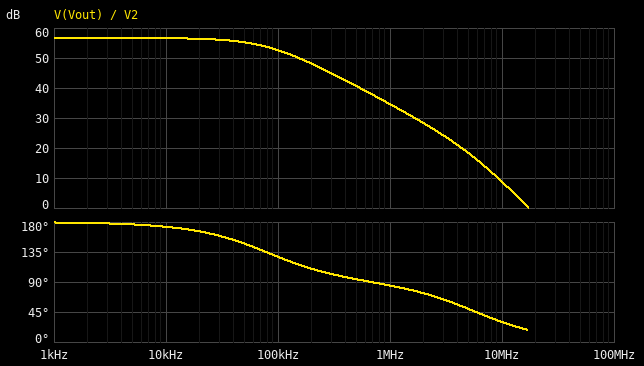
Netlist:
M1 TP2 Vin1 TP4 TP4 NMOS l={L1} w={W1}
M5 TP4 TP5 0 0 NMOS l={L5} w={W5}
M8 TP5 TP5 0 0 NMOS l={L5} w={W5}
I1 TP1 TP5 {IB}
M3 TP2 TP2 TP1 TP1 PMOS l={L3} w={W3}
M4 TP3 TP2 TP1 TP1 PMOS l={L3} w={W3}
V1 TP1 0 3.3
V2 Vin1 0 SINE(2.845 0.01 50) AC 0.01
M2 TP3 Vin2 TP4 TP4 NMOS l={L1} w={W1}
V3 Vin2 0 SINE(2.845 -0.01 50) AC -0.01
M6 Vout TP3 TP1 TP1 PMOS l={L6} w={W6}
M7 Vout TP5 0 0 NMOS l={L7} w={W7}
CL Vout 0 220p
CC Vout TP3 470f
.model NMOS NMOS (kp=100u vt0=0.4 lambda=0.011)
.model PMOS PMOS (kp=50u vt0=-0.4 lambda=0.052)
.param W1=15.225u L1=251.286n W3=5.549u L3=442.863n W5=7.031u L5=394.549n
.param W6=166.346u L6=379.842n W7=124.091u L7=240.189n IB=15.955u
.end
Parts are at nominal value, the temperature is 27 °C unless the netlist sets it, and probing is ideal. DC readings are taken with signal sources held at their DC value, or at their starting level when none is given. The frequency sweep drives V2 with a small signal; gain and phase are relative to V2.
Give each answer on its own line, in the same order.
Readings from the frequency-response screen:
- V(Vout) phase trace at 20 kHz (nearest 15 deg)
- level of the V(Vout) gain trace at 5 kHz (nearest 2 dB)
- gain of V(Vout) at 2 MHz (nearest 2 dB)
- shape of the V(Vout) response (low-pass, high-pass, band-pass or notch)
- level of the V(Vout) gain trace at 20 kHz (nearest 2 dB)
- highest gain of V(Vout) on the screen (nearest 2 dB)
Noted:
165 deg
56 dB
28 dB
low-pass
56 dB
56 dB
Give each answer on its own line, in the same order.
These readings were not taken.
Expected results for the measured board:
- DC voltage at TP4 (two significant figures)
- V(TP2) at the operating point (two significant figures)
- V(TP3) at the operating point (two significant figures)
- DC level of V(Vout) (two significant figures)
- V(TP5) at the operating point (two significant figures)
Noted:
2.4 V
2.7 V
2.7 V
61 mV
530 mV
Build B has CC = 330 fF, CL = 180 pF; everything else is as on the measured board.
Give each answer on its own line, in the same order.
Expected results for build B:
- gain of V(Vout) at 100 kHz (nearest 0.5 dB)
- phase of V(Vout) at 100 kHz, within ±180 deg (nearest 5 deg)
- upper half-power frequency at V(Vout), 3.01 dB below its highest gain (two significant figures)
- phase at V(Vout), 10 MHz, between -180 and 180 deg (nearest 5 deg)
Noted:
54.0 dB
140 deg
110 kHz
35 deg
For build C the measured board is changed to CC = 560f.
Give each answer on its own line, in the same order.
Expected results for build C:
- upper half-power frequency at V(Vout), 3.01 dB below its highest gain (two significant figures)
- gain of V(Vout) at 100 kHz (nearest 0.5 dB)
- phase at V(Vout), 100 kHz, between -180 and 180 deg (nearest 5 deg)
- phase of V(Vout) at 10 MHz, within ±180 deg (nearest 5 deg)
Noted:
68 kHz
51.5 dB
125 deg
30 deg
